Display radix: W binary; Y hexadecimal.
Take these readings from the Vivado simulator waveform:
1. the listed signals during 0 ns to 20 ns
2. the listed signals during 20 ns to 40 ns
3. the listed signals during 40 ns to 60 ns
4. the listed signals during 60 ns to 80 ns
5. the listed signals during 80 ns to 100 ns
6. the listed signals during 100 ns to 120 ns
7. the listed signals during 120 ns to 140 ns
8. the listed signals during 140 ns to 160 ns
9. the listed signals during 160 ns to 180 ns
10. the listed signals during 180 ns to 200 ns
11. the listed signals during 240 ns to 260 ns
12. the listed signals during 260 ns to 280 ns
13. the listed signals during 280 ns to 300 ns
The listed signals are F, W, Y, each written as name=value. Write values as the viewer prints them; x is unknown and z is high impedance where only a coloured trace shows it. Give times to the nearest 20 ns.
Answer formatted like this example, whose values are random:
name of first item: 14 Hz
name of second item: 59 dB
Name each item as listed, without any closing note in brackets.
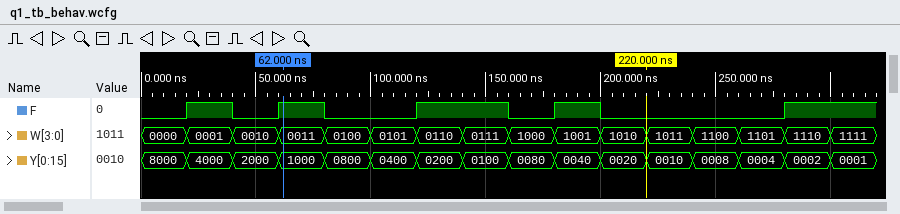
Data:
the listed signals during 0 ns to 20 ns: F=0, W=0000, Y=8000
the listed signals during 20 ns to 40 ns: F=1, W=0001, Y=4000
the listed signals during 40 ns to 60 ns: F=0, W=0010, Y=2000
the listed signals during 60 ns to 80 ns: F=1, W=0011, Y=1000
the listed signals during 80 ns to 100 ns: F=0, W=0100, Y=0800
the listed signals during 100 ns to 120 ns: F=0, W=0101, Y=0400
the listed signals during 120 ns to 140 ns: F=1, W=0110, Y=0200
the listed signals during 140 ns to 160 ns: F=1, W=0111, Y=0100
the listed signals during 160 ns to 180 ns: F=0, W=1000, Y=0080
the listed signals during 180 ns to 200 ns: F=1, W=1001, Y=0040
the listed signals during 240 ns to 260 ns: F=0, W=1100, Y=0008
the listed signals during 260 ns to 280 ns: F=0, W=1101, Y=0004
the listed signals during 280 ns to 300 ns: F=1, W=1110, Y=0002
